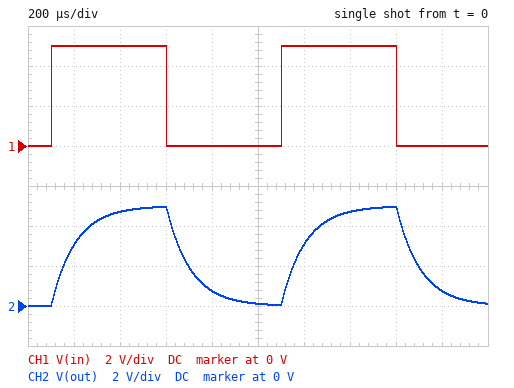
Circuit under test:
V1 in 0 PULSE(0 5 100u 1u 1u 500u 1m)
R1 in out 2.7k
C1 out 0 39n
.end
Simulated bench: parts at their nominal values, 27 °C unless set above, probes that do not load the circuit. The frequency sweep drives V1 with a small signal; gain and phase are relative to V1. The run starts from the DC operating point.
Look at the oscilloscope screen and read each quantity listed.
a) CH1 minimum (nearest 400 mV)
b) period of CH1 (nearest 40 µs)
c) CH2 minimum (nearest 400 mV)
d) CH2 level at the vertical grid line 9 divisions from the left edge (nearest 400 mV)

0 V
1.00 ms
0 V
800 mV
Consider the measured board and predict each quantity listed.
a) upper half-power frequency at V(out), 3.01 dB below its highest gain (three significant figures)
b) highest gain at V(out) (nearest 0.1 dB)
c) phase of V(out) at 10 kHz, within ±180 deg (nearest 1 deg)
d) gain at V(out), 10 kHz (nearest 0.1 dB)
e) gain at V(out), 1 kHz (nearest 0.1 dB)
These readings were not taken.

1.51 kHz
0 dB
-81 deg
-16.5 dB
-1.6 dB
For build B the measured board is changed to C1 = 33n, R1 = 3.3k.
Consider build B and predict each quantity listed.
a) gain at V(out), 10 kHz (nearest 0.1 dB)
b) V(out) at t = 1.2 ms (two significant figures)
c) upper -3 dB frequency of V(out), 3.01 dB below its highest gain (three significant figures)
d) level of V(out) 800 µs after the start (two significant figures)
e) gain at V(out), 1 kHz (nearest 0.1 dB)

-16.8 dB
3.0 V
1.46 kHz
800 mV
-1.7 dB
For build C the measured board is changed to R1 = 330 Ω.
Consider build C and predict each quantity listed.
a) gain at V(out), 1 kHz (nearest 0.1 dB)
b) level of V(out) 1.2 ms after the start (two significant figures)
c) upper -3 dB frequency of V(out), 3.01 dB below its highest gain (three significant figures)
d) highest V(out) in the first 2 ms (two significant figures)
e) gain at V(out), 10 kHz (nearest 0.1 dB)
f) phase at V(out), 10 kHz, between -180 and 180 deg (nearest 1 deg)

0 dB
5.0 V
12.4 kHz
5.0 V
-2.2 dB
-39 deg
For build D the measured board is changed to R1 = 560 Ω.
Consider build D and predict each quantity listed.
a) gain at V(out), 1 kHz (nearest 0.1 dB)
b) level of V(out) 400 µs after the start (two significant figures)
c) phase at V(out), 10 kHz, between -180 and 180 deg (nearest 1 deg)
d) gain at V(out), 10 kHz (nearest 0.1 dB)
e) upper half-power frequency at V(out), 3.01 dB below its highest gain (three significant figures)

-0.1 dB
5.0 V
-54 deg
-4.6 dB
7.29 kHz
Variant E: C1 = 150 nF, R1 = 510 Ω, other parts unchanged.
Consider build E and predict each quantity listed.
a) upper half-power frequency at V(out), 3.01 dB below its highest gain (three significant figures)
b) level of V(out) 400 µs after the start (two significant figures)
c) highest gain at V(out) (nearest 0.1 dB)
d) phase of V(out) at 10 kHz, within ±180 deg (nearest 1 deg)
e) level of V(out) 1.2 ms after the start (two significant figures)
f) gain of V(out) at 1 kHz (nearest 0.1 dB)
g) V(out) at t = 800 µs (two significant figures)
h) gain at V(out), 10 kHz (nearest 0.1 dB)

2.08 kHz
4.9 V
0 dB
-78 deg
3.6 V
-0.9 dB
370 mV
-13.8 dB
